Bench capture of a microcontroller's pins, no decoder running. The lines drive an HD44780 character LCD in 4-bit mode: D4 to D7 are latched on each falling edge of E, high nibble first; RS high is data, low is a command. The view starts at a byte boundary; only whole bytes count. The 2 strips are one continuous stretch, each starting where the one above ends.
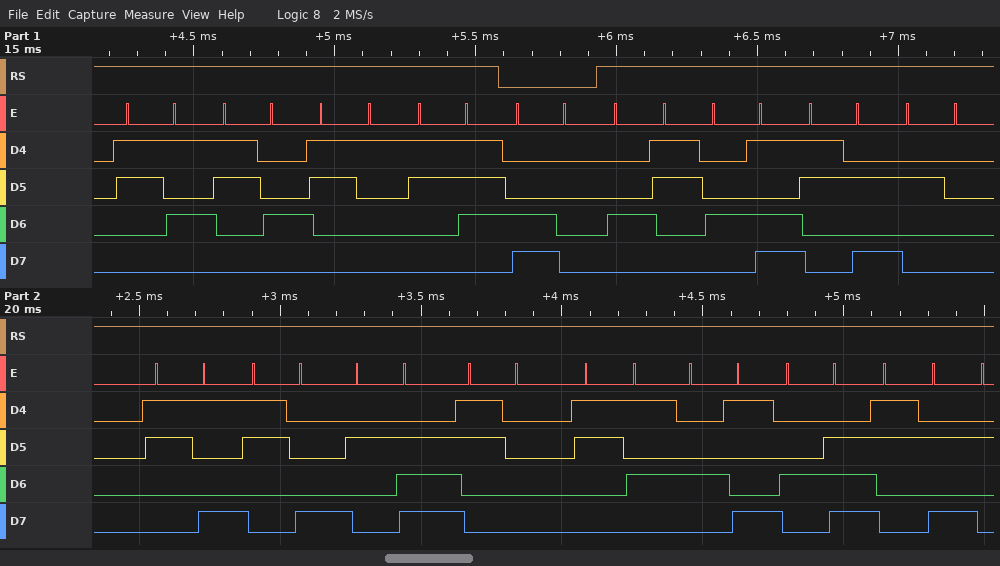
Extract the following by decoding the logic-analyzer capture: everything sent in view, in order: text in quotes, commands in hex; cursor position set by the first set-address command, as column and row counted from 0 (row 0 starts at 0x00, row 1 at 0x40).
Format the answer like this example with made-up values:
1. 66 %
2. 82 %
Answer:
1. "5417" 0xC0 "CM: 98.05IN:"
2. column 0, row 1
